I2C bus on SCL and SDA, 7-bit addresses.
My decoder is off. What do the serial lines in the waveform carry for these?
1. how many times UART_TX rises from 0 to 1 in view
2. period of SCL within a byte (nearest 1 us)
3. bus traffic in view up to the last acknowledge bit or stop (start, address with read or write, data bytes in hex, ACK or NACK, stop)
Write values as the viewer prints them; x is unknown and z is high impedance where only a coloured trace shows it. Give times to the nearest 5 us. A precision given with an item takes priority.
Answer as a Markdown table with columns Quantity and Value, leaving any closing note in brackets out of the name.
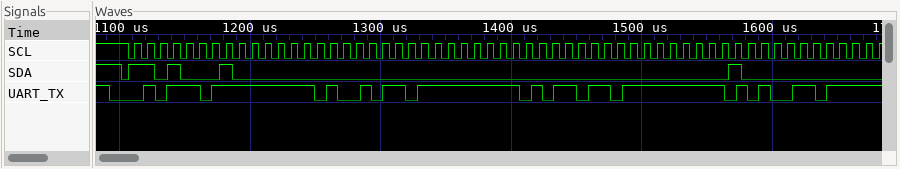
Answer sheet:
| Quantity | Value |
|---|---|
| how many times UART_TX rises from 0 to 1 in view | 15 |
| period of SCL within a byte | 10 us |
| bus traffic in view up to the last acknowledge bit or stop | start, address 68 read ACK, 00 ACK, 00 ACK, 00 ACK, 00 ACK, 40 ACK |
